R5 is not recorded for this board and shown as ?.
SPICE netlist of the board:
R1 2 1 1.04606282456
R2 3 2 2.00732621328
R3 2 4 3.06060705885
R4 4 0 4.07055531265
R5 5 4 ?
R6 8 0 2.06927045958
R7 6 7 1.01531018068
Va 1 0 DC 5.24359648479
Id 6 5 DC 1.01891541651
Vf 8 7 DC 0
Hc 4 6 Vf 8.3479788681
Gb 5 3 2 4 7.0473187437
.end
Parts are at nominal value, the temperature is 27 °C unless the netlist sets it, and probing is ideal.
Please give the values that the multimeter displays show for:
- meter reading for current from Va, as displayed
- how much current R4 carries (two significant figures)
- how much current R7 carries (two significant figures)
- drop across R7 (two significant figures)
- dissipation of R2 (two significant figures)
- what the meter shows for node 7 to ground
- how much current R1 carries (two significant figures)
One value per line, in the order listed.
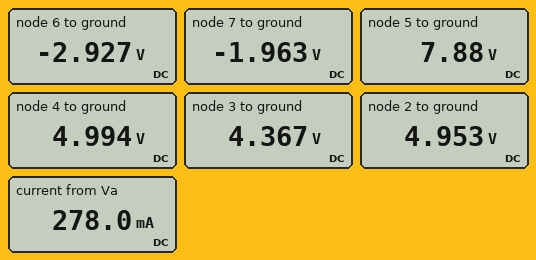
278.0 mA
1.2 A
950 mA
960 mV
170 mW
-1.963 V
280 mA
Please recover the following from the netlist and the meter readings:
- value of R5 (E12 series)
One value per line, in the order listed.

2.2 Ω
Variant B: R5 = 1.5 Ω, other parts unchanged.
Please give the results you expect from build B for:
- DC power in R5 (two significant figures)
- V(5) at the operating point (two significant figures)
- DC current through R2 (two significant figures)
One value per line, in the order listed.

2.6 W
7.0 V
290 mA
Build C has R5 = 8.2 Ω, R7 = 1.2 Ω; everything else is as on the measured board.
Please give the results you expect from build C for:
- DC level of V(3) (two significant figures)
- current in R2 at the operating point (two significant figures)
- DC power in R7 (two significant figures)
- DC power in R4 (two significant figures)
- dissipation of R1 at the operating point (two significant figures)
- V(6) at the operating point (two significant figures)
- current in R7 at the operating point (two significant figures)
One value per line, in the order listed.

4.5 V
260 mA
1.2 W
6.2 W
63 mW
-3.2 V
990 mA
